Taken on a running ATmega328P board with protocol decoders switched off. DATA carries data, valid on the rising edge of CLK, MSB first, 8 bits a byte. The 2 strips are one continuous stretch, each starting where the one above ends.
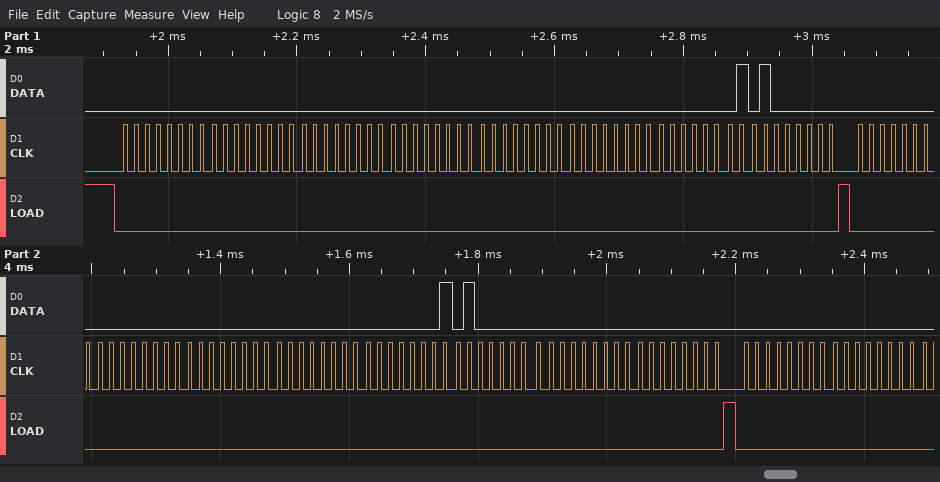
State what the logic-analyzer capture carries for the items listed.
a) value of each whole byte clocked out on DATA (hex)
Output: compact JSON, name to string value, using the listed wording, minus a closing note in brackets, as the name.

{"value of each whole byte clocked out on DATA": "00 00 00 00 00 00 01 40 00 00 00 00 01 40 00 00 00 00"}
